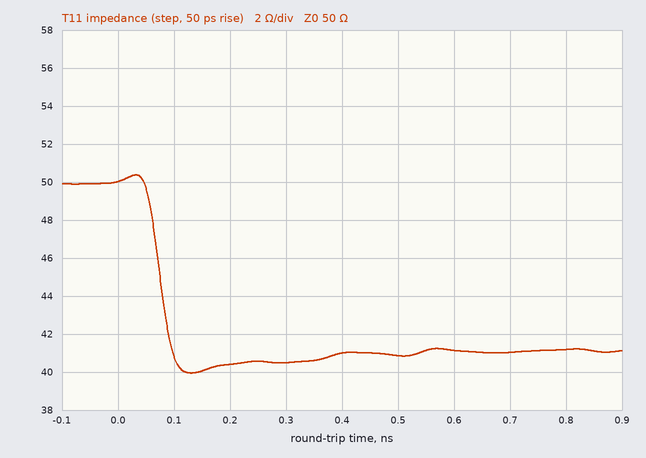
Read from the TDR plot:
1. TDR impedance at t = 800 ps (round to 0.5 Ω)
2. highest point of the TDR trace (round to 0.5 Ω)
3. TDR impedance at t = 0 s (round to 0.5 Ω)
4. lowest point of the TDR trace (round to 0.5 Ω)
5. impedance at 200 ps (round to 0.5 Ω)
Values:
41.0 Ω
50.5 Ω
50.0 Ω
40.0 Ω
40.5 Ω
